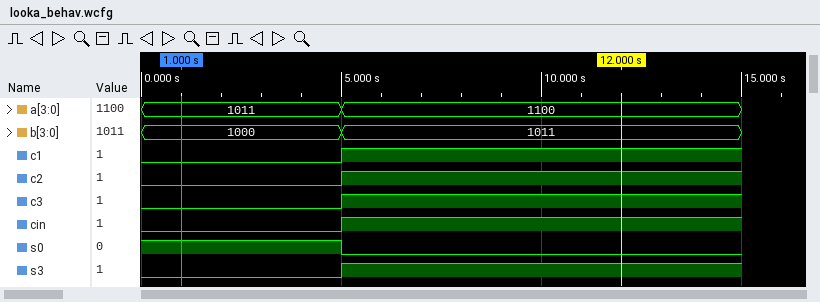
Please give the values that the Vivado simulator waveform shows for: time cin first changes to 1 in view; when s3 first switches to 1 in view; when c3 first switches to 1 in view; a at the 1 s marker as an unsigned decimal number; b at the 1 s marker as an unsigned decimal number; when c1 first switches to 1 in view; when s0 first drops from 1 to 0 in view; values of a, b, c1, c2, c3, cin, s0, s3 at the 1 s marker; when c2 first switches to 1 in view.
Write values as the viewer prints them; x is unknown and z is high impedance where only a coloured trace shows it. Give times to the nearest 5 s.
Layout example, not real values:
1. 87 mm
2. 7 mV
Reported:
1. 5 s
2. 5 s
3. 5 s
4. 11
5. 8
6. 5 s
7. 5 s
8. a=1011, b=1000, c1=0, c2=0, c3=0, cin=0, s0=1, s3=0
9. 5 s
